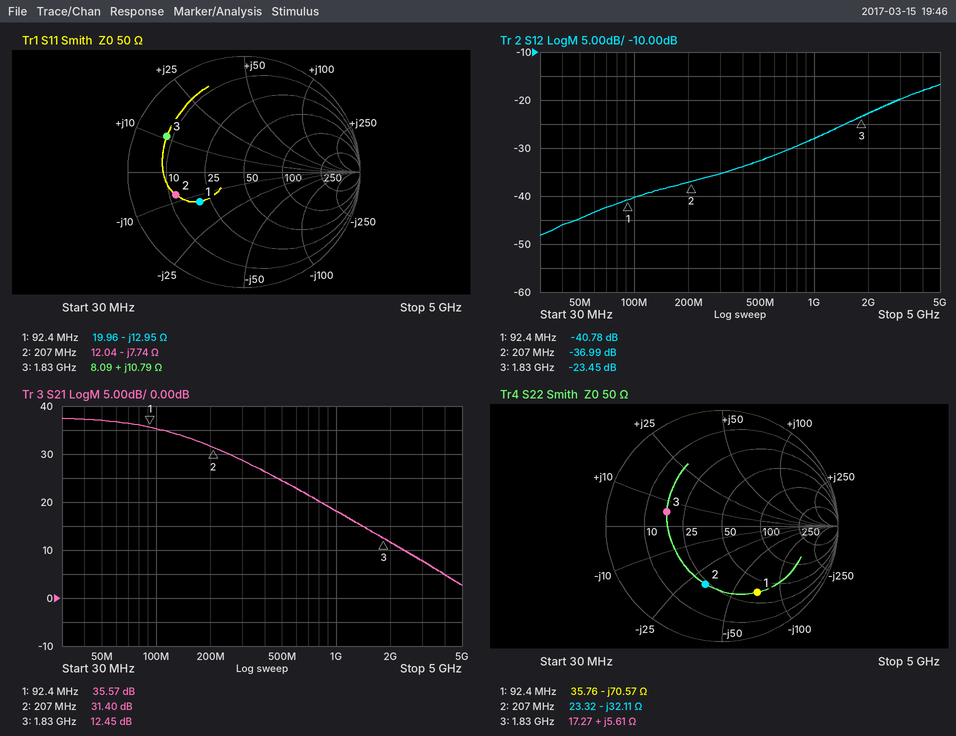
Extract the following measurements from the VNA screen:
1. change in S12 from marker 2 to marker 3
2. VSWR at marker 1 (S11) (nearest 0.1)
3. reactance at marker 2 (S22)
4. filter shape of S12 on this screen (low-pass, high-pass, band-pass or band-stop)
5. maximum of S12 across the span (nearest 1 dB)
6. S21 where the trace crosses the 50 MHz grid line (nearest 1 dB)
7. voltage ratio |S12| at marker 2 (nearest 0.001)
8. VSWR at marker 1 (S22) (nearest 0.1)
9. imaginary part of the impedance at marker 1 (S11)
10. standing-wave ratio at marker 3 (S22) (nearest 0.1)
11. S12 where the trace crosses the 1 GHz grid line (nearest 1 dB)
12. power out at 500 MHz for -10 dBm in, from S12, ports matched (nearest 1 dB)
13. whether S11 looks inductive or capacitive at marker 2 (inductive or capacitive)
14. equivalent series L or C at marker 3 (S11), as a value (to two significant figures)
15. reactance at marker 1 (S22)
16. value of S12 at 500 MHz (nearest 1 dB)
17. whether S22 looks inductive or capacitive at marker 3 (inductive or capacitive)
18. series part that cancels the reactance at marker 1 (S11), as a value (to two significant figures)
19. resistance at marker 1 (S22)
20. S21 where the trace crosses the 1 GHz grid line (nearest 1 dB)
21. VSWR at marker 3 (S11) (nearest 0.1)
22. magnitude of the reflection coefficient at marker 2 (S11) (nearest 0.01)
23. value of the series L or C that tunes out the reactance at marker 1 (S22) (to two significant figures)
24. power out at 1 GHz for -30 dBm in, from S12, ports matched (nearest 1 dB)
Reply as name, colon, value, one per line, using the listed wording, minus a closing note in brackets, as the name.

change in S12 from marker 2 to marker 3: 13.54 dB
VSWR at marker 1 (S11): 2.7
reactance at marker 2: -32.11 Ω
filter shape of S12 on this screen: high-pass
maximum of S12 across the span: -17 dB
S21 where the trace crosses the 50 MHz grid line: 37 dB
voltage ratio |S12| at marker 2: 0.014
VSWR at marker 1 (S22): 4.7
imaginary part of the impedance at marker 1: -12.95 Ω
standing-wave ratio at marker 3 (S22): 2.9
S12 where the trace crosses the 1 GHz grid line: -28 dB
power out at 500 MHz for -10 dBm in, from S12, ports matched: -43 dBm
whether S11 looks inductive or capacitive at marker 2: capacitive
equivalent series L or C at marker 3 (S11), as a value: 940 pH
reactance at marker 1: -70.57 Ω
value of S12 at 500 MHz: -33 dB
whether S22 looks inductive or capacitive at marker 3: inductive
series part that cancels the reactance at marker 1 (S11), as a value: 22 nH
resistance at marker 1: 35.76 Ω
S21 where the trace crosses the 1 GHz grid line: 18 dB
VSWR at marker 3 (S11): 6.5
magnitude of the reflection coefficient at marker 2 (S11): 0.62
value of the series L or C that tunes out the reactance at marker 1 (S22): 120 nH
power out at 1 GHz for -30 dBm in, from S12, ports matched: -58 dBm
